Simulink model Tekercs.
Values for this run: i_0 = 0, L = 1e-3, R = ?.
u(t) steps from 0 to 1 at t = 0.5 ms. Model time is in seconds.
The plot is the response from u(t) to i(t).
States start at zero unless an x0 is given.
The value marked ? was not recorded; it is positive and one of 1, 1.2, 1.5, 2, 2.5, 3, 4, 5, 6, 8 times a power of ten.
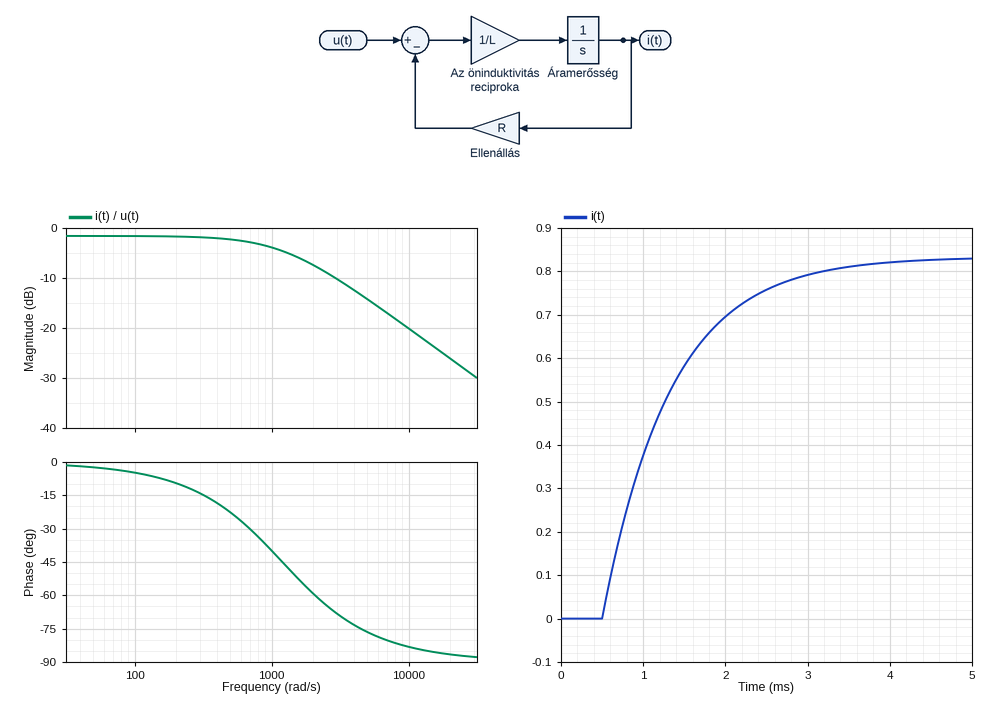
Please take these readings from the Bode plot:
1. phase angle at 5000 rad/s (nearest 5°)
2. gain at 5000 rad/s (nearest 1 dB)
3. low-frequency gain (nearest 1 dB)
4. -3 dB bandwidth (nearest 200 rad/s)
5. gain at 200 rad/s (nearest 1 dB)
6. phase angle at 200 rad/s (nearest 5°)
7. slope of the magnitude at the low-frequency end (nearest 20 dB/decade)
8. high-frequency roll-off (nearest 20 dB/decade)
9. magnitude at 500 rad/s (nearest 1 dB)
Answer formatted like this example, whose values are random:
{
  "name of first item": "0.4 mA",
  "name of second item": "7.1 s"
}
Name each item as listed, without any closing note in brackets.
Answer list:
{
  "phase angle at 5000 rad/s": "-75°",
  "gain at 5000 rad/s": "-14 dB",
  "low-frequency gain": "-2 dB",
  "-3 dB bandwidth": "1200 rad/s",
  "gain at 200 rad/s": "-2 dB",
  "phase angle at 200 rad/s": "-10°",
  "slope of the magnitude at the low-frequency end": "0 dB/decade",
  "high-frequency roll-off": "-20 dB/decade",
  "magnitude at 500 rad/s": "-2 dB"
}
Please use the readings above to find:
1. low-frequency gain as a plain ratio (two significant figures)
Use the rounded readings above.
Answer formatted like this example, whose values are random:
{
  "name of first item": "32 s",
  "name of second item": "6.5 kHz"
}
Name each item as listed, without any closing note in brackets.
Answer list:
{
  "low-frequency gain as a plain ratio": "0.79"
}
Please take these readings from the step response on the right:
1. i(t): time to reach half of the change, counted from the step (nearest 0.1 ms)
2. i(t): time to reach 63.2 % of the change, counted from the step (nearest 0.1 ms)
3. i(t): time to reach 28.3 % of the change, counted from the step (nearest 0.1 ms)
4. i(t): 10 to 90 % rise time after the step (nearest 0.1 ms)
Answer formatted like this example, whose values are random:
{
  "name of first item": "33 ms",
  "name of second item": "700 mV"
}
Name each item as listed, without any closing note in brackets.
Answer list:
{
  "i(t): time to reach half of the change, counted from the step": "0.6 ms",
  "i(t): time to reach 63.2 % of the change, counted from the step": "0.8 ms",
  "i(t): time to reach 28.3 % of the change, counted from the step": "0.3 ms",
  "i(t): 10 to 90 % rise time after the step": "1.8 ms"
}
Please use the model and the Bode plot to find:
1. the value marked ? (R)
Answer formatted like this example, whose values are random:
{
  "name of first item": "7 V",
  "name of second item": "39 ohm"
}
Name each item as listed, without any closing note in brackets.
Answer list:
{
  "the value marked ?": "1.2"
}
